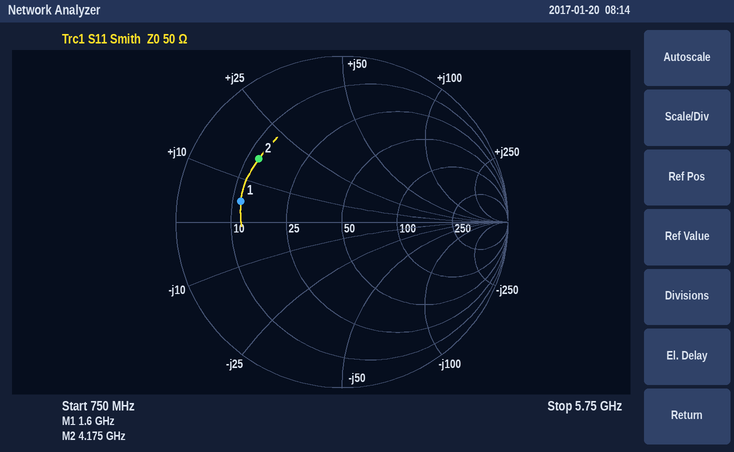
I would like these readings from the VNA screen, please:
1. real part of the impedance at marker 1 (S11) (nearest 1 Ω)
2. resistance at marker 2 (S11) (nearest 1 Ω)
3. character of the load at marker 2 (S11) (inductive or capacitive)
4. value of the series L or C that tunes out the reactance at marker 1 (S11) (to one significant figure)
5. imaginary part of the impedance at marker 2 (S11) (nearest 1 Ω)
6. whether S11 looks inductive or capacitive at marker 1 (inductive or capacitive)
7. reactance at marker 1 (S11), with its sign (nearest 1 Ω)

12 Ω
13 Ω
inductive
20 pF
+16 Ω
inductive
+5 Ω
